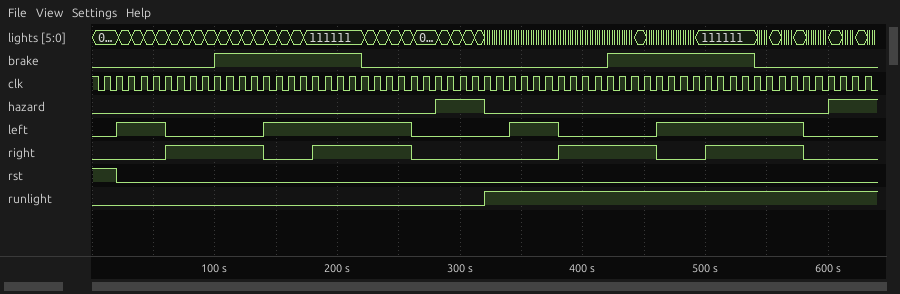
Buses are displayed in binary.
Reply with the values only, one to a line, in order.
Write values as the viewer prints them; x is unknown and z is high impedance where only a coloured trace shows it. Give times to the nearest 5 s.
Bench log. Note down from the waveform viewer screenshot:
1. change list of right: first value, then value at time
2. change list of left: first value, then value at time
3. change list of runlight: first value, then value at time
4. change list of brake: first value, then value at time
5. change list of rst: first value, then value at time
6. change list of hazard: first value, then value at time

0, 1 at 60 s, 0 at 140 s, 1 at 180 s, 0 at 260 s, 1 at 380 s, 0 at 460 s, 1 at 500 s, 0 at 580 s
0, 1 at 20 s, 0 at 60 s, 1 at 140 s, 0 at 260 s, 1 at 340 s, 0 at 380 s, 1 at 460 s, 0 at 580 s
0, 1 at 320 s
0, 1 at 100 s, 0 at 220 s, 1 at 420 s, 0 at 540 s
1, 0 at 20 s
0, 1 at 280 s, 0 at 320 s, 1 at 600 s
